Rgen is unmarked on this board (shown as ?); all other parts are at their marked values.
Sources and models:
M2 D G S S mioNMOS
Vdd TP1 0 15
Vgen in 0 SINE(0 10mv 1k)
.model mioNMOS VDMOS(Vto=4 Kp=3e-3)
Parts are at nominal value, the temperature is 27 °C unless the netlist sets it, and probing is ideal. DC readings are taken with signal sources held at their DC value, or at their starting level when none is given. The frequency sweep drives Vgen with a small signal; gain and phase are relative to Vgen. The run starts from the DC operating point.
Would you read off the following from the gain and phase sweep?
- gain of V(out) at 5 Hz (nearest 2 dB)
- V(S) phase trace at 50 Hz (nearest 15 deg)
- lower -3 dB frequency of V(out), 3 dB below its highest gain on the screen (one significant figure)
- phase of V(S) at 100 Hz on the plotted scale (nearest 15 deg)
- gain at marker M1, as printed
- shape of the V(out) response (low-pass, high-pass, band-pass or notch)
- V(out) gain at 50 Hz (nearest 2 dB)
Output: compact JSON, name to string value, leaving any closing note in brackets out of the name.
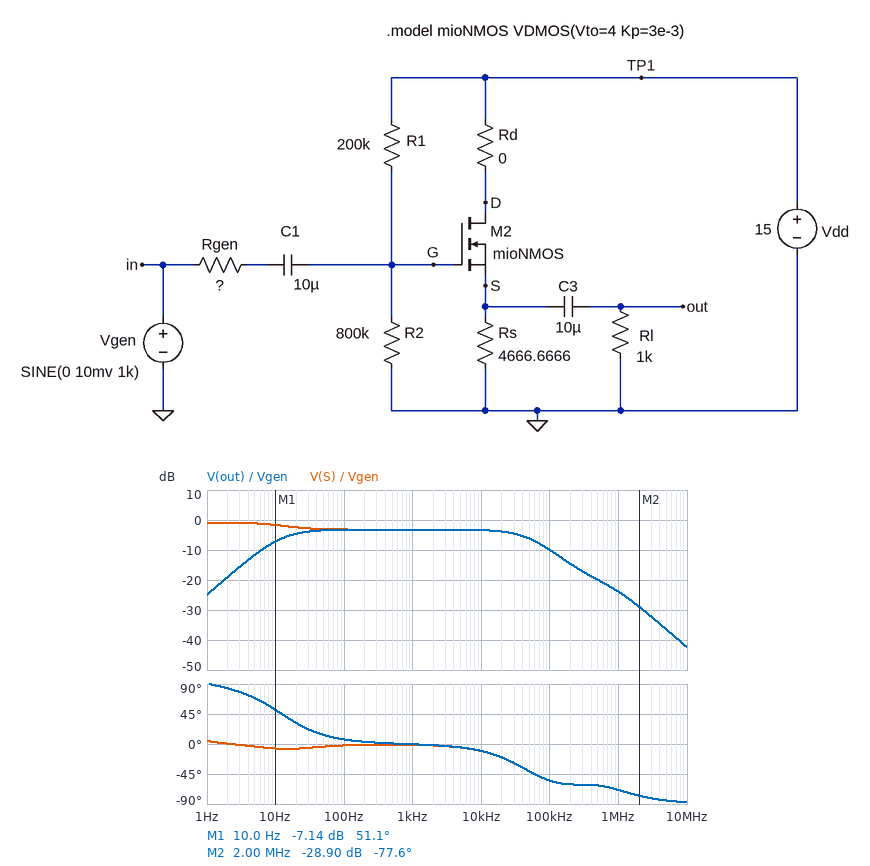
{"gain of V(out) at 5 Hz": "-12 dB", "V(S) phase trace at 50 Hz": "0 deg", "lower -3 dB frequency of V(out), 3 dB below its highest gain on the screen": "10 Hz", "phase of V(S) at 100 Hz on the plotted scale": "0 deg", "gain at marker M1, as printed": "-7.14 dB", "shape of the V(out) response": "band-pass", "V(out) gain at 50 Hz": "-4 dB"}
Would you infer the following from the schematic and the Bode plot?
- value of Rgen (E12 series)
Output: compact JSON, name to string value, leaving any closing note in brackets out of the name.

{"value of Rgen": "4.7 kΩ"}
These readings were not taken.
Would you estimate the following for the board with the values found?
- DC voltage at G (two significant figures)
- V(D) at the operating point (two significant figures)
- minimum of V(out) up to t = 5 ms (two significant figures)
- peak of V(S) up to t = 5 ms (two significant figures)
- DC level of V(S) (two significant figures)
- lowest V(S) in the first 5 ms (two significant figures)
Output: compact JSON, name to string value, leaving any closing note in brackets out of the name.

{"DC voltage at G": "12 V", "V(D) at the operating point": "15 V", "minimum of V(out) up to t = 5 ms": "-7.0 mV", "peak of V(S) up to t = 5 ms": "7.0 V", "DC level of V(S)": "7.0 V", "lowest V(S) in the first 5 ms": "7.0 V"}
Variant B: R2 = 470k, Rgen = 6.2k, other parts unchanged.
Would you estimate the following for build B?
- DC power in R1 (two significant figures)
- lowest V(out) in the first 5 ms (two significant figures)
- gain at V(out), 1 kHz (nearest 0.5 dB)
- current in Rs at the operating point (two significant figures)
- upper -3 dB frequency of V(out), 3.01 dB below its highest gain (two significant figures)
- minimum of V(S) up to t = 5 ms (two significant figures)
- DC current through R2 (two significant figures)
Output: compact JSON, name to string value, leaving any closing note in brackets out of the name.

{"DC power in R1": "100 µW", "lowest V(out) in the first 5 ms": "-6.7 mV", "gain at V(out), 1 kHz": "-3.5 dB", "current in Rs at the operating point": "1.2 mA", "upper -3 dB frequency of V(out), 3.01 dB below its highest gain": "41 kHz", "minimum of V(S) up to t = 5 ms": "5.6 V", "DC current through R2": "22 µA"}
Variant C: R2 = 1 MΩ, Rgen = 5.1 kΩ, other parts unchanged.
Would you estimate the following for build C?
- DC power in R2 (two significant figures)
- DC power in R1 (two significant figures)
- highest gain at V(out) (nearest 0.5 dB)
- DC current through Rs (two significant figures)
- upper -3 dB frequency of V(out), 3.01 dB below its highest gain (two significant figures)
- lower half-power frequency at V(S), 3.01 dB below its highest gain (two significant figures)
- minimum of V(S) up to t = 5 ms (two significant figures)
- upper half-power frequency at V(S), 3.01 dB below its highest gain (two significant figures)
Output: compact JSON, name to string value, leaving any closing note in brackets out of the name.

{"DC power in R2": "160 µW", "DC power in R1": "31 µW", "highest gain at V(out)": "-3.0 dB", "DC current through Rs": "1.6 mA", "upper -3 dB frequency of V(out), 3.01 dB below its highest gain": "44 kHz", "lower half-power frequency at V(S), 3.01 dB below its highest gain": "92 mHz", "minimum of V(S) up to t = 5 ms": "7.5 V", "upper half-power frequency at V(S), 3.01 dB below its highest gain": "19 kHz"}
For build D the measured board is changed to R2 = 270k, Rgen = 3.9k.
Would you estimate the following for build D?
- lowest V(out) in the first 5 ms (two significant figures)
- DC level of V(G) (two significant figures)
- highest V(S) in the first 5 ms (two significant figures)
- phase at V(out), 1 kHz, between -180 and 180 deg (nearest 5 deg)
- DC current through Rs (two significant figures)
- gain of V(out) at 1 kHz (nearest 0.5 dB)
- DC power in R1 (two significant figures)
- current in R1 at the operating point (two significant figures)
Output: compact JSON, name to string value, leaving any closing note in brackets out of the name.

{"lowest V(out) in the first 5 ms": "-6.3 mV", "DC level of V(G)": "8.6 V", "highest V(S) in the first 5 ms": "3.9 V", "phase at V(out), 1 kHz, between -180 and 180 deg": "0 deg", "DC current through Rs": "830 µA", "gain of V(out) at 1 kHz": "-4.0 dB", "DC power in R1": "200 µW", "current in R1 at the operating point": "32 µA"}
